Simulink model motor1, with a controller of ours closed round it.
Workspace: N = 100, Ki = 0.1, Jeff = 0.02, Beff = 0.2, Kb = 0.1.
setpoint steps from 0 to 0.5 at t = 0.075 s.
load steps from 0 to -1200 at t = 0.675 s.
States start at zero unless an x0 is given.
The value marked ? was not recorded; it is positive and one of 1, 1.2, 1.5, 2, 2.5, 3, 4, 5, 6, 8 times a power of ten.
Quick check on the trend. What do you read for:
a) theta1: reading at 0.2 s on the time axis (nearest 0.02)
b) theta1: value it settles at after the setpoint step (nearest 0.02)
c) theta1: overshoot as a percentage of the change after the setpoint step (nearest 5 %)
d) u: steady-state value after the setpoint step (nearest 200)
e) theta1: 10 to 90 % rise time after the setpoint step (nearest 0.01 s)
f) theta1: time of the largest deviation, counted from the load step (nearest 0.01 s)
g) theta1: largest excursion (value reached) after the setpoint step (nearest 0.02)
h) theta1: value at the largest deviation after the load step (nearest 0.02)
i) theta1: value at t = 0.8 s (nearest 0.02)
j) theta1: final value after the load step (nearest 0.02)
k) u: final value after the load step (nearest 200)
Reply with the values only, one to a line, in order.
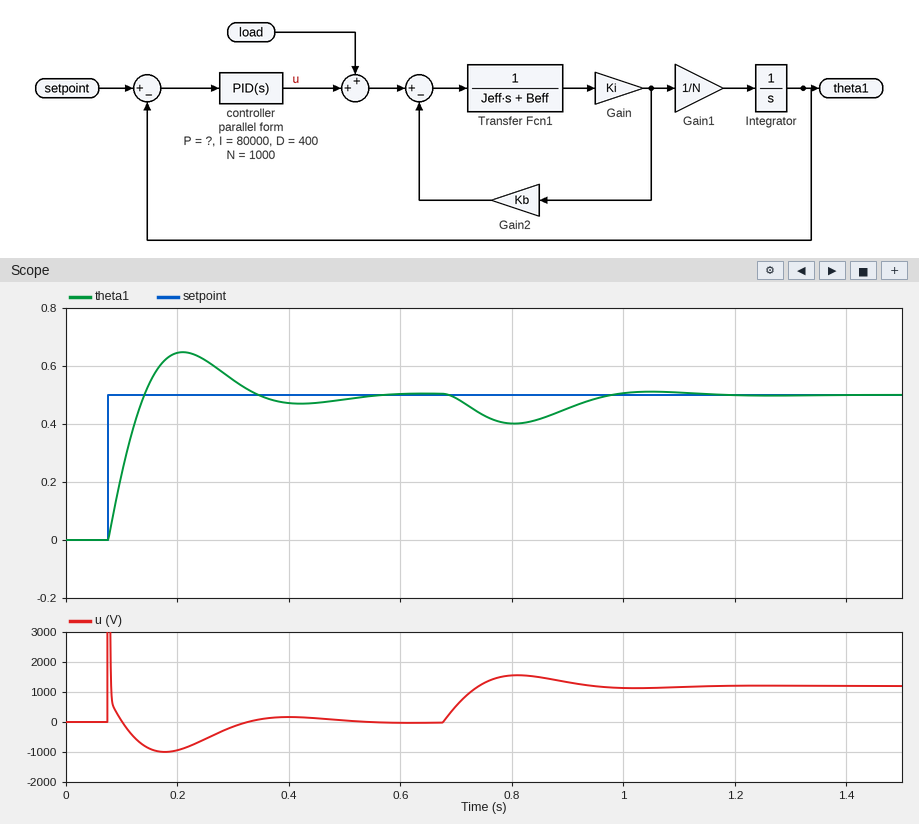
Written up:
0.64
0.50
30 %
0
0.05 s
0.13 s
0.64
0.40
0.40
0.50
1200
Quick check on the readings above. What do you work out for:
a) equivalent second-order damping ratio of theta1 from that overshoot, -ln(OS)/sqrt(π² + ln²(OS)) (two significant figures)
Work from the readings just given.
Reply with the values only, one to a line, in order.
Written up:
0.36
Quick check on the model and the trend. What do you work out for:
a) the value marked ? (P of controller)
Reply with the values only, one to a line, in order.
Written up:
10000
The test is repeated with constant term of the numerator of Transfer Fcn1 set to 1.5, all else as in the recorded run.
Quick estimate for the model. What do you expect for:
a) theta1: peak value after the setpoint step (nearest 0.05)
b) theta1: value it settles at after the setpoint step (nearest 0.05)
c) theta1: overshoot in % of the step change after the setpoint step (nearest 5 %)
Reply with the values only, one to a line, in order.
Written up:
0.60
0.50
25 %
